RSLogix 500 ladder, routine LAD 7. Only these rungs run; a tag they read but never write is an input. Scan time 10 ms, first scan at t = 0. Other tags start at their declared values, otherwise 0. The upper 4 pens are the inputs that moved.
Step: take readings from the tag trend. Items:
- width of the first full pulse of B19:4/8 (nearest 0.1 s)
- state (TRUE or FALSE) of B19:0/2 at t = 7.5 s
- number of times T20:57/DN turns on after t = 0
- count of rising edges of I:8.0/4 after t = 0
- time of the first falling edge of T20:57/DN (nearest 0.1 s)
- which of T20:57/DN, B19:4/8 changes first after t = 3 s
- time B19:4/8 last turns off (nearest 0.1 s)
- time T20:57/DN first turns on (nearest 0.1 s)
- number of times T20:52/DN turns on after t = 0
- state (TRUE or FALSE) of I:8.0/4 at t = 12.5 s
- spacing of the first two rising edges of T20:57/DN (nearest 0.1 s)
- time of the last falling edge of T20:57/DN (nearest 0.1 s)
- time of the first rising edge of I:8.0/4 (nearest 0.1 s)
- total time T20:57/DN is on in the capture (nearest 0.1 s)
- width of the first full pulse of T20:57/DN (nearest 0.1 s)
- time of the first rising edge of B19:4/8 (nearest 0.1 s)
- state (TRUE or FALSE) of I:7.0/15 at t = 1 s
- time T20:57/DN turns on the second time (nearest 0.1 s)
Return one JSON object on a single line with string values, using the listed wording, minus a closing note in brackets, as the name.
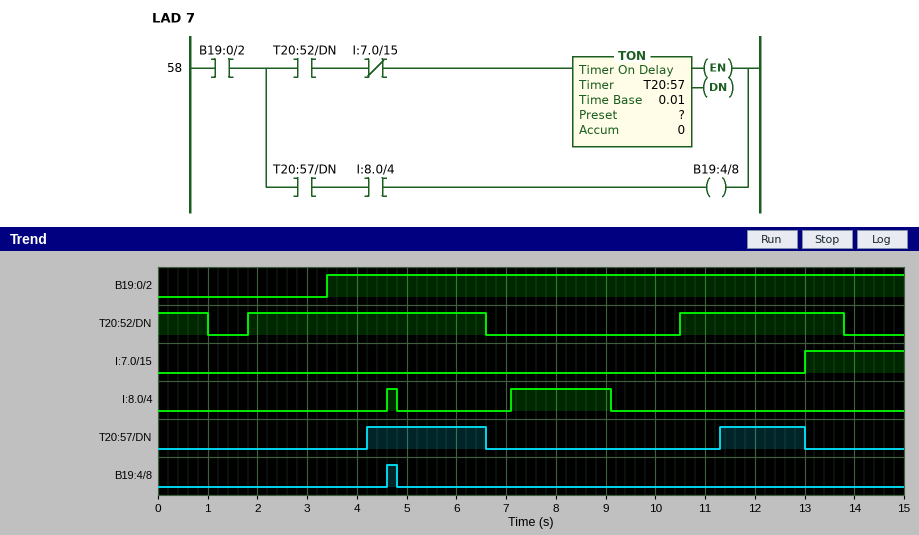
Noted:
{"width of the first full pulse of B19:4/8": "0.2 s", "state (TRUE or FALSE) of B19:0/2 at t = 7.5 s": "TRUE", "number of times T20:57/DN turns on after t = 0": "2", "count of rising edges of I:8.0/4 after t = 0": "2", "time of the first falling edge of T20:57/DN": "6.6 s", "which of T20:57/DN, B19:4/8 changes first after t = 3 s": "T20:57/DN", "time B19:4/8 last turns off": "4.8 s", "time T20:57/DN first turns on": "4.2 s", "number of times T20:52/DN turns on after t = 0": "2", "state (TRUE or FALSE) of I:8.0/4 at t = 12.5 s": "FALSE", "spacing of the first two rising edges of T20:57/DN": "7.1 s", "time of the last falling edge of T20:57/DN": "13.0 s", "time of the first rising edge of I:8.0/4": "4.6 s", "total time T20:57/DN is on in the capture": "4.1 s", "width of the first full pulse of T20:57/DN": "2.4 s", "time of the first rising edge of B19:4/8": "4.6 s", "state (TRUE or FALSE) of I:7.0/15 at t = 1 s": "FALSE", "time T20:57/DN turns on the second time": "11.3 s"}
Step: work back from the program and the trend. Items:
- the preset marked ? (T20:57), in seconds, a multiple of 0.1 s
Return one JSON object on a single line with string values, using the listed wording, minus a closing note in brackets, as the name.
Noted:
{"the preset marked ? (T20:57), in seconds, a multiple of 0.1 s": "0.8 s"}
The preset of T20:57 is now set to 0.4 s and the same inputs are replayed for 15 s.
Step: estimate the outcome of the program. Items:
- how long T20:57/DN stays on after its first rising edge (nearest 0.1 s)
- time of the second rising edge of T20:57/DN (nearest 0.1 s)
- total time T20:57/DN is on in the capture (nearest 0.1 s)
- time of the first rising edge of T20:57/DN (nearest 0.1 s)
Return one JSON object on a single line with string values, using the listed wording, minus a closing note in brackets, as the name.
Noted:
{"how long T20:57/DN stays on after its first rising edge": "2.8 s", "time of the second rising edge of T20:57/DN": "10.9 s", "total time T20:57/DN is on in the capture": "4.9 s", "time of the first rising edge of T20:57/DN": "3.8 s"}
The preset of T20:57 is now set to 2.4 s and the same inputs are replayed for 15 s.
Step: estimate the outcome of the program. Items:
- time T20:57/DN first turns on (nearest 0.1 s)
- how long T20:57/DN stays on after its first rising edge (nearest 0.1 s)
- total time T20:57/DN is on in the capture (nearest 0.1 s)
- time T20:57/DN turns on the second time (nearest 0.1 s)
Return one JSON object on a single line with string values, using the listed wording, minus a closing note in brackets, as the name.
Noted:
{"time T20:57/DN first turns on": "5.8 s", "how long T20:57/DN stays on after its first rising edge": "0.8 s", "total time T20:57/DN is on in the capture": "0.9 s", "time T20:57/DN turns on the second time": "12.9 s"}
